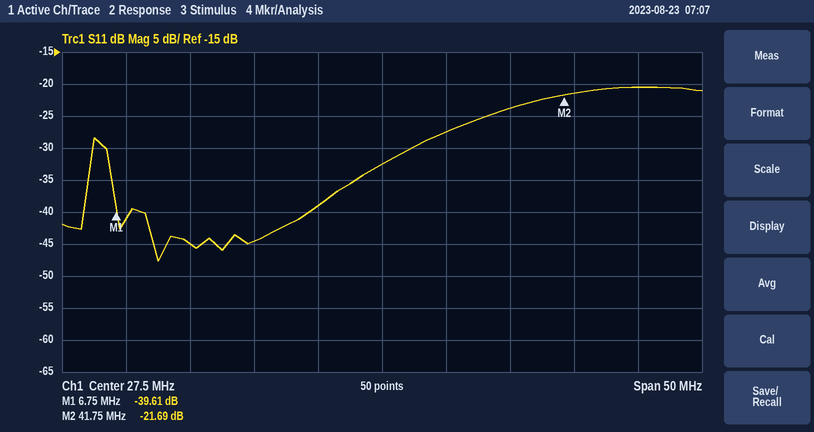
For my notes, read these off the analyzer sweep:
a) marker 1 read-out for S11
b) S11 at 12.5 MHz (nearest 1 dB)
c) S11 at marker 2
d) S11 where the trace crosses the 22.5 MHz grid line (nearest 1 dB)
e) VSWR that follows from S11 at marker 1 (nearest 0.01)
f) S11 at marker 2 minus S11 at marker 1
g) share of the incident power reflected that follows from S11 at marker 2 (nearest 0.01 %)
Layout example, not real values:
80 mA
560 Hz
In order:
-39.61 dB
-45 dB
-21.69 dB
-39 dB
1.02
17.92 dB
0.68 %
